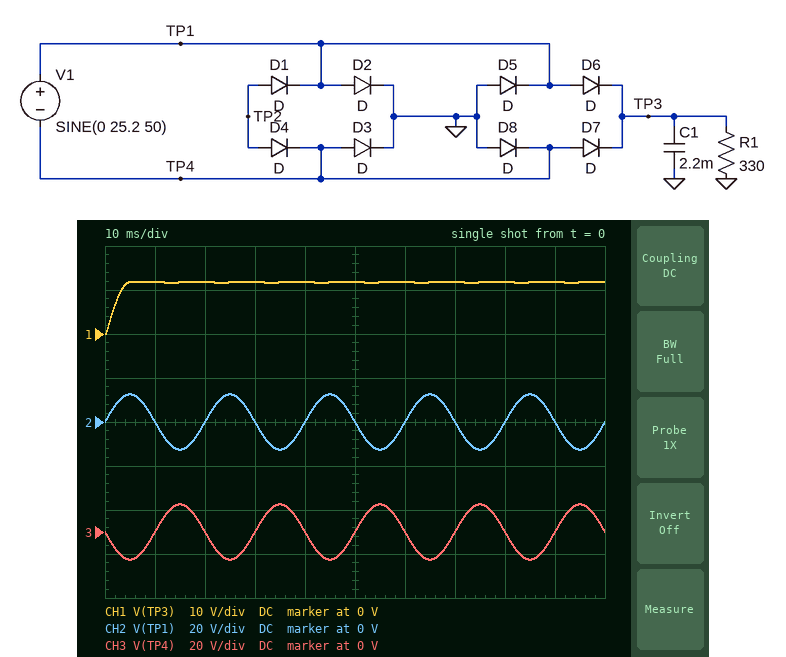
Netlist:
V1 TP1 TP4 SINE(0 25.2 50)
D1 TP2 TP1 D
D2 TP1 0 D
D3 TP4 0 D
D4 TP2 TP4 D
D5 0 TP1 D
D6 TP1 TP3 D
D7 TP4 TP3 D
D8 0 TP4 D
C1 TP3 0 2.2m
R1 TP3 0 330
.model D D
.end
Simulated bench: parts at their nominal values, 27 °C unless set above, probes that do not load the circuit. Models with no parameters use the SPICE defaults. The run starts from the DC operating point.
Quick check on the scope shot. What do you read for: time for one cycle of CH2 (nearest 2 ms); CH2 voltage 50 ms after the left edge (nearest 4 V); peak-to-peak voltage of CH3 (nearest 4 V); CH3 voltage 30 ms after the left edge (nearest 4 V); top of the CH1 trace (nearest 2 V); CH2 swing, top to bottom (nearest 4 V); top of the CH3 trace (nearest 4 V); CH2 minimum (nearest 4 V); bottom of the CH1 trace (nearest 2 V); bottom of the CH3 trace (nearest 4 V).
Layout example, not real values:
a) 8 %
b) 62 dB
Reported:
a) 20 ms
b) 0 V
c) 24 V
d) 0 V
e) 12 V
f) 24 V
g) 12 V
h) -12 V
i) 0 V
j) -12 V
